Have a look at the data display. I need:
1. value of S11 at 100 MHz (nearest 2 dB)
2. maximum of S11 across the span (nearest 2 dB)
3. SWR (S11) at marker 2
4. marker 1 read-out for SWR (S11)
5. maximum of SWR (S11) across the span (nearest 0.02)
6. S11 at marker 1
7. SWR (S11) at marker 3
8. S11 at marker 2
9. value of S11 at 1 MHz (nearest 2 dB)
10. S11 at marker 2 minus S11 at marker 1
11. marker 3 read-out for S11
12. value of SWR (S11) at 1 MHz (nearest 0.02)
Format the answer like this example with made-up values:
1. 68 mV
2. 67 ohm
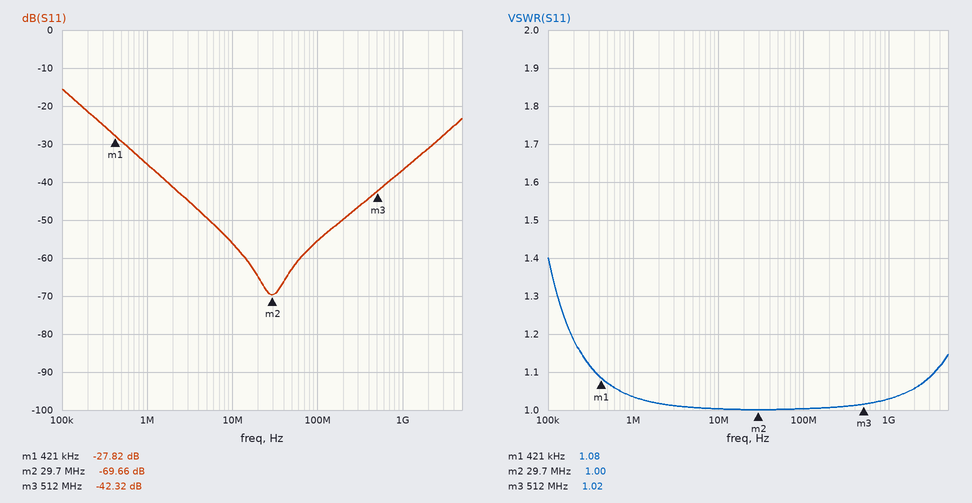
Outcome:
1. -56 dB
2. -16 dB
3. 1.00
4. 1.08
5. 1.40
6. -27.82 dB
7. 1.02
8. -69.66 dB
9. -36 dB
10. -41.84 dB
11. -42.32 dB
12. 1.04
